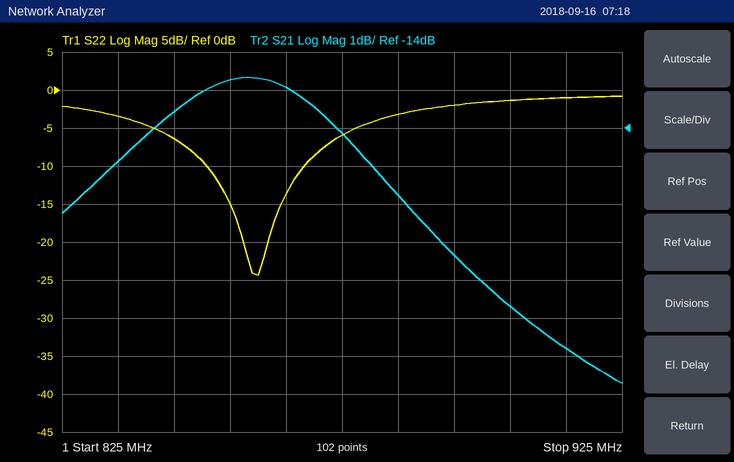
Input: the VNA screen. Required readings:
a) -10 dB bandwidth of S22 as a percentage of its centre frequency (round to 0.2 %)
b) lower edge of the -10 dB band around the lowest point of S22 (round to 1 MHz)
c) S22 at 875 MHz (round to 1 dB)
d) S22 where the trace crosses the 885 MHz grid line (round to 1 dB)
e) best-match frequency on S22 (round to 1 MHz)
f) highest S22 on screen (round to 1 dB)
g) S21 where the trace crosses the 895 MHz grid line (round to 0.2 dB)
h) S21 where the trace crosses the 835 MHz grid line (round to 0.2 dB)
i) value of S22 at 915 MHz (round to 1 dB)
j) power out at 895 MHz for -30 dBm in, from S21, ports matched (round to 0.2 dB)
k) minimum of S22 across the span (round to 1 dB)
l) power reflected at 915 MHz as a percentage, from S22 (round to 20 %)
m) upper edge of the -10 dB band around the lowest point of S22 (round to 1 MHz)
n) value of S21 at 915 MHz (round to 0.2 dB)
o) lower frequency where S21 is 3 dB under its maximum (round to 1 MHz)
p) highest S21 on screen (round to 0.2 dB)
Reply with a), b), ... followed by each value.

a) 2.0 %
b) 851 MHz
c) -6 dB
d) -3 dB
e) 860 MHz
f) -1 dB
g) -17.4 dB
h) -14.8 dB
i) -1 dB
j) -47.4 dBm
k) -24 dB
l) 80 %
m) 868 MHz
n) -19.8 dB
o) 829 MHz
p) -12.6 dB
